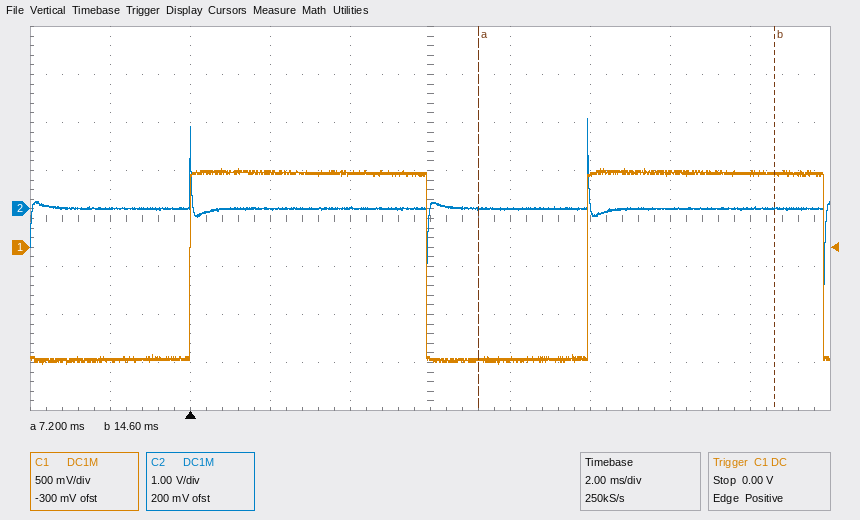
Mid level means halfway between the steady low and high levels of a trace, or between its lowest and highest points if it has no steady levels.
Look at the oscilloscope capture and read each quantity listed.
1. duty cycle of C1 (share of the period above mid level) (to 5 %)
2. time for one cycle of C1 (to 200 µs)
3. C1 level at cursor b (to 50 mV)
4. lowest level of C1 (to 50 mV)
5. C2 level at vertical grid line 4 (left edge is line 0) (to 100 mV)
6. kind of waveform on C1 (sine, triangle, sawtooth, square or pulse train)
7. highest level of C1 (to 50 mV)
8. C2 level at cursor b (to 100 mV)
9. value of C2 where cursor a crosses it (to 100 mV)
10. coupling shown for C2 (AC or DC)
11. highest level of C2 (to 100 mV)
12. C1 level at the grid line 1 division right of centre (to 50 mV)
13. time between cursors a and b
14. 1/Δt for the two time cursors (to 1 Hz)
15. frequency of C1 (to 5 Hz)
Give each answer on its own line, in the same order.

60 %
10.0 ms
750 mV
-1.20 V
0.0 V
pulse train
800 mV
0.0 V
0.0 V
DC
1.9 V
-1.15 V
7.4 ms
135 Hz
100 Hz
